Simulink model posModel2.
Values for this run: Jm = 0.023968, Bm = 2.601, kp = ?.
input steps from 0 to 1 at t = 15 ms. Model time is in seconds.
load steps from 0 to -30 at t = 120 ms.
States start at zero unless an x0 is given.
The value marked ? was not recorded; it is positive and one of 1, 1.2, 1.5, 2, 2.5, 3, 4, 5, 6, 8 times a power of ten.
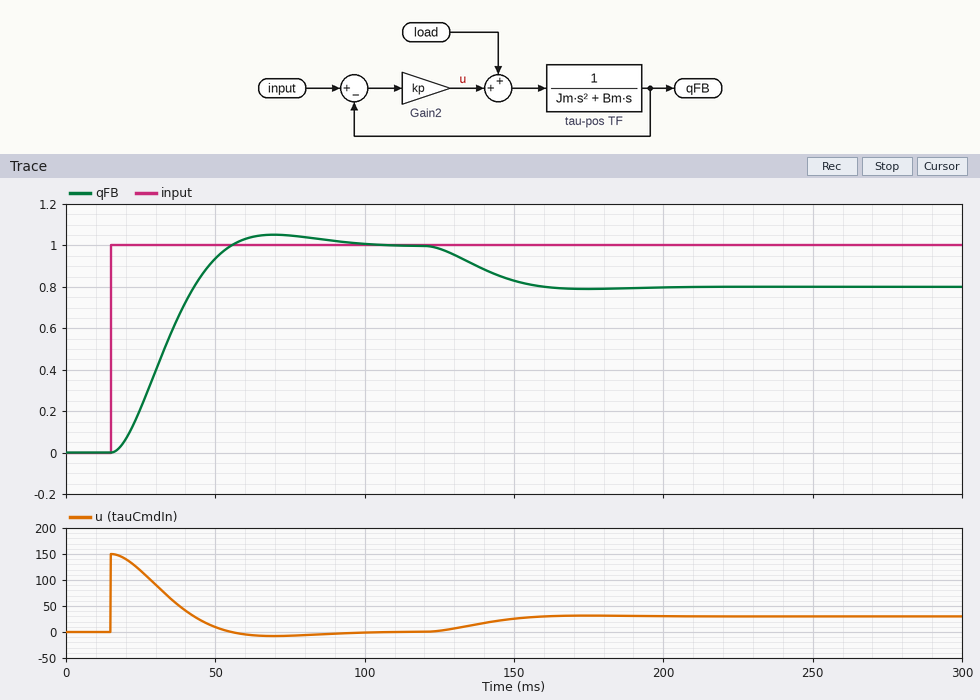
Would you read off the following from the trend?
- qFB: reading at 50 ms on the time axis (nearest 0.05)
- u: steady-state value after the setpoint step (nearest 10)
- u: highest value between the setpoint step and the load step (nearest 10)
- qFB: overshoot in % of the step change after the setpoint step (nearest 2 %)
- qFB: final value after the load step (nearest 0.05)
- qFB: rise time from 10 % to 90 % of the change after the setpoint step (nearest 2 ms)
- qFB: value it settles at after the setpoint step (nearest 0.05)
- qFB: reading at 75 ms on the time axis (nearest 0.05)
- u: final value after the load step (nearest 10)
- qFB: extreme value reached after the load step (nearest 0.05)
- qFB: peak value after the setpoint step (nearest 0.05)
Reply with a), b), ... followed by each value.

a) 0.95
b) 0
c) 150
d) 6 %
e) 0.80
f) 26 ms
g) 1.00
h) 1.05
i) 30
j) 0.80
k) 1.05
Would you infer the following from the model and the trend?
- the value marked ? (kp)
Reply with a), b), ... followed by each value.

a) 150
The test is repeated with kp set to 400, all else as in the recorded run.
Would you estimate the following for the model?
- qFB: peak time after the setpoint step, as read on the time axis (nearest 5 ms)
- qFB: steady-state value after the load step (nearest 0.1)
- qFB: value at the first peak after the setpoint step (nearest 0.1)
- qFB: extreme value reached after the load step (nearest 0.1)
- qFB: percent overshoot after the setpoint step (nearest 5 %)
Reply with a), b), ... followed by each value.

a) 40 ms
b) 0.9
c) 1.2
d) 0.9
e) 25 %
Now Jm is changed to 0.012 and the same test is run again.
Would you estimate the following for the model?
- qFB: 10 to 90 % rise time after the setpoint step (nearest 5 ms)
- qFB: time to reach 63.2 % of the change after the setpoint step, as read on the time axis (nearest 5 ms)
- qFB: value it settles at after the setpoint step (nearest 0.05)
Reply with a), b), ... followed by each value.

a) 30 ms
b) 35 ms
c) 1.00
